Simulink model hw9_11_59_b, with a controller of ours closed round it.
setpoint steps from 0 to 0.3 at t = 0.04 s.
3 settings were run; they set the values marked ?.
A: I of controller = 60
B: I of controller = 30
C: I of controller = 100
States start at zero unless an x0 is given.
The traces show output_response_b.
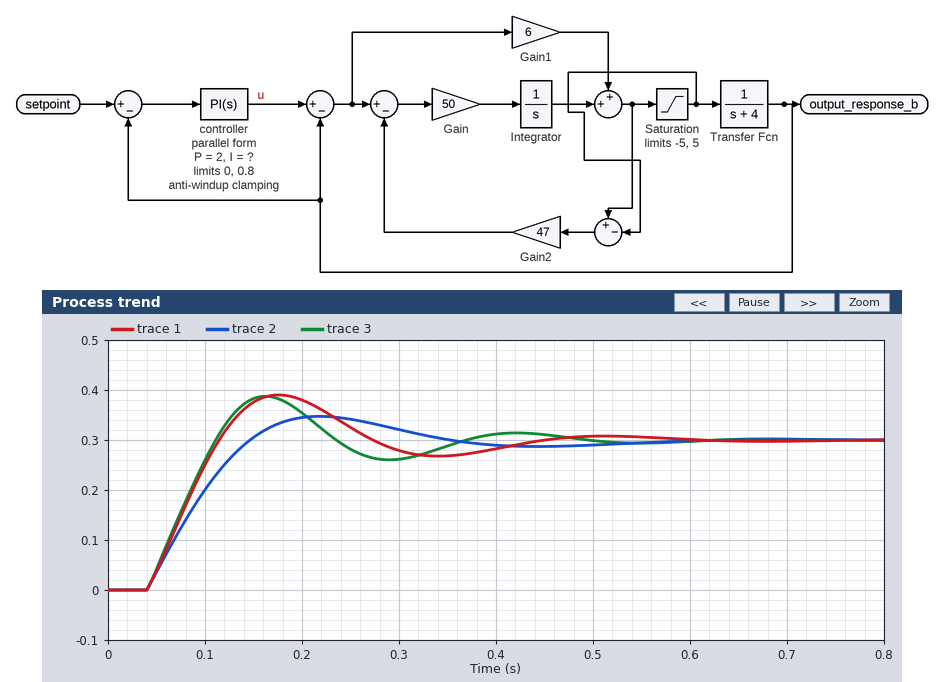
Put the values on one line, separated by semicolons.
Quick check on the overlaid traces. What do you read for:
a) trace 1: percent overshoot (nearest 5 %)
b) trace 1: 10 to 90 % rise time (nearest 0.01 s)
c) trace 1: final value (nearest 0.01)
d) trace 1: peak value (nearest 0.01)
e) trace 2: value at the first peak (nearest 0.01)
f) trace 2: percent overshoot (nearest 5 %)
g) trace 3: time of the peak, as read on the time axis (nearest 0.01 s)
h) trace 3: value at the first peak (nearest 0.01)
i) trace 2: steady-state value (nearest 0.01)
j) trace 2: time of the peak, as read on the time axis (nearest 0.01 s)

30 %; 0.06 s; 0.30; 0.39; 0.35; 15 %; 0.16 s; 0.39; 0.30; 0.22 s
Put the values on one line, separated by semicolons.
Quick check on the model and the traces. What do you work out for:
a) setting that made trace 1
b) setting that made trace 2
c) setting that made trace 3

A; B; C
